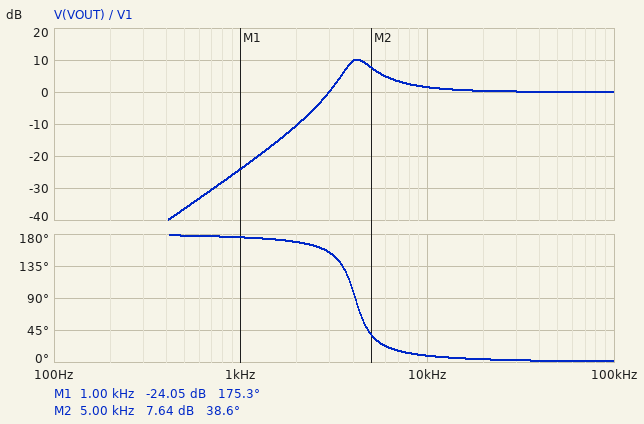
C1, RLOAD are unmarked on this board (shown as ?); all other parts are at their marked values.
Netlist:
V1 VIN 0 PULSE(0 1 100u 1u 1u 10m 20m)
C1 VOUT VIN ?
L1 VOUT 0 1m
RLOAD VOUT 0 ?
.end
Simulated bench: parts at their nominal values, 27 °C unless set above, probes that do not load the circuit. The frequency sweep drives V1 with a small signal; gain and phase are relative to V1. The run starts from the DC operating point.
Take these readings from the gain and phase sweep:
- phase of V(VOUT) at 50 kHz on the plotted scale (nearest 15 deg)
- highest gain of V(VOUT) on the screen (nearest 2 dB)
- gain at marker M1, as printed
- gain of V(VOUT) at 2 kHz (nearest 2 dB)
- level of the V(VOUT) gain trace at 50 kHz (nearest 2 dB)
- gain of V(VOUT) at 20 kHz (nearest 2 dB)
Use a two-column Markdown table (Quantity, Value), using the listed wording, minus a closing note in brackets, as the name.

| Quantity | Value |
|---|---|
| phase of V(VOUT) at 50 kHz on the plotted scale | 0 deg |
| highest gain of V(VOUT) on the screen | 10 dB |
| gain at marker M1, as printed | -24.05 dB |
| gain of V(VOUT) at 2 kHz | -10 dB |
| level of the V(VOUT) gain trace at 50 kHz | 0 dB |
| gain of V(VOUT) at 20 kHz | 0 dB |
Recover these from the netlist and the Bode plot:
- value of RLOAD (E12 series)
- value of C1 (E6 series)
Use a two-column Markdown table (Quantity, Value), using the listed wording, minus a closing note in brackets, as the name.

| Quantity | Value |
|---|---|
| value of RLOAD | 82 Ω |
| value of C1 | 1.5 µF |
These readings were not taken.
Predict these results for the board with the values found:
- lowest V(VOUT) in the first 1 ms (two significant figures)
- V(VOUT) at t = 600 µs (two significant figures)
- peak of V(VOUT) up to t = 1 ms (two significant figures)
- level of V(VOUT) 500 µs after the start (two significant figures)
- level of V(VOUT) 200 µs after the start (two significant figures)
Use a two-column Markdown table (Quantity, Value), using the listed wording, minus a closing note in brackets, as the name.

| Quantity | Value |
|---|---|
| lowest V(VOUT) in the first 1 ms | -640 mV |
| V(VOUT) at t = 600 µs | 130 mV |
| peak of V(VOUT) up to t = 1 ms | 1.0 V |
| level of V(VOUT) 500 µs after the start | -120 mV |
| level of V(VOUT) 200 µs after the start | -610 mV |
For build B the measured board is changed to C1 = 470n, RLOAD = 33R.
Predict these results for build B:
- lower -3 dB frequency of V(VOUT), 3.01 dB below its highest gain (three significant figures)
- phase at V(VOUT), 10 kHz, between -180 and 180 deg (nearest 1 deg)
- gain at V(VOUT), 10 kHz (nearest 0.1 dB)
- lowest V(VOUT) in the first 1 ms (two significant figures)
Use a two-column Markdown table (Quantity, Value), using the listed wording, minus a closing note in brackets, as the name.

| Quantity | Value |
|---|---|
| lower -3 dB frequency of V(VOUT), 3.01 dB below its highest gain | 7.26 kHz |
| phase at V(VOUT), 10 kHz, between -180 and 180 deg | 66 deg |
| gain at V(VOUT), 10 kHz | -1.0 dB |
| lowest V(VOUT) in the first 1 ms | -210 mV |
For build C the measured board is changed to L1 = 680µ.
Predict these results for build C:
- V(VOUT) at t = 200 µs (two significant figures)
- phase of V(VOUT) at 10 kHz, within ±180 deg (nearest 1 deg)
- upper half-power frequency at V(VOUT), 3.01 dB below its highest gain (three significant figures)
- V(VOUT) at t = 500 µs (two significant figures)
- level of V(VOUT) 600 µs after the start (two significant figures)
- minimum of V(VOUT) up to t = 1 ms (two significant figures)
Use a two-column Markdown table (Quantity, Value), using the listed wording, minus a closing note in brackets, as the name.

| Quantity | Value |
|---|---|
| V(VOUT) at t = 200 µs | -670 mV |
| phase of V(VOUT) at 10 kHz, within ±180 deg | 10 deg |
| upper half-power frequency at V(VOUT), 3.01 dB below its highest gain | 5.92 kHz |
| V(VOUT) at t = 500 µs | 200 mV |
| level of V(VOUT) 600 µs after the start | -130 mV |
| minimum of V(VOUT) up to t = 1 ms | -690 mV |
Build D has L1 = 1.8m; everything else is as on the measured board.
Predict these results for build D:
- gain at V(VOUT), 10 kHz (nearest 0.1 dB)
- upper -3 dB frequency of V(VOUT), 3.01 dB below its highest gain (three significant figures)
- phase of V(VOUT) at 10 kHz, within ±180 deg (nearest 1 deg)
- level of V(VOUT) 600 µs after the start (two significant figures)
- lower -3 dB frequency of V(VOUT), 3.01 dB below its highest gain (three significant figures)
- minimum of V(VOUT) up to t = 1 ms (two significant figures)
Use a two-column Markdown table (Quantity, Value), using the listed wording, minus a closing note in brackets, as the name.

| Quantity | Value |
|---|---|
| gain at V(VOUT), 10 kHz | 0.8 dB |
| upper -3 dB frequency of V(VOUT), 3.01 dB below its highest gain | 4.34 kHz |
| phase of V(VOUT) at 10 kHz, within ±180 deg | 8 deg |
| level of V(VOUT) 600 µs after the start | -130 mV |
| lower -3 dB frequency of V(VOUT), 3.01 dB below its highest gain | 2.66 kHz |
| minimum of V(VOUT) up to t = 1 ms | -560 mV |
